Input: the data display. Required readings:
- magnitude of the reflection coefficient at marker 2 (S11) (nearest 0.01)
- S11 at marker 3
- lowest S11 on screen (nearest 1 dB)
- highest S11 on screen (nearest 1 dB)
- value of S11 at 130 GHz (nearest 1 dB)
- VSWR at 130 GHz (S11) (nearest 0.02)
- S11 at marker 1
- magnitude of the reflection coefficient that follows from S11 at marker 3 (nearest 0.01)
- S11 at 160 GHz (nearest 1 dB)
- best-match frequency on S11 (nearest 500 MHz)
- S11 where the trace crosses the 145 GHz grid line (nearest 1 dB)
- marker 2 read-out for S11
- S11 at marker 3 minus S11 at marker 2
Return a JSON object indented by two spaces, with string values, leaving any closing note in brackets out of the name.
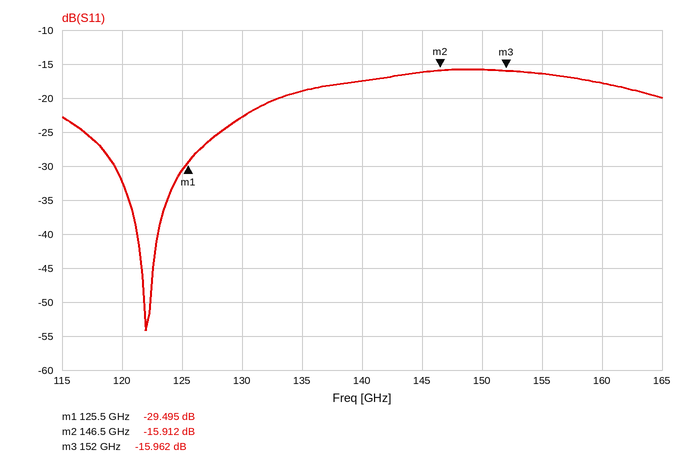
{
  "magnitude of the reflection coefficient at marker 2 (S11)": "0.16",
  "S11 at marker 3": "-15.962 dB",
  "lowest S11 on screen": "-54 dB",
  "highest S11 on screen": "-16 dB",
  "value of S11 at 130 GHz": "-23 dB",
  "VSWR at 130 GHz (S11)": "1.16",
  "S11 at marker 1": "-29.495 dB",
  "magnitude of the reflection coefficient that follows from S11 at marker 3": "0.16",
  "S11 at 160 GHz": "-18 dB",
  "best-match frequency on S11": "122.0 GHz",
  "S11 where the trace crosses the 145 GHz grid line": "-16 dB",
  "marker 2 read-out for S11": "-15.912 dB",
  "S11 at marker 3 minus S11 at marker 2": "-0.050 dB"
}
